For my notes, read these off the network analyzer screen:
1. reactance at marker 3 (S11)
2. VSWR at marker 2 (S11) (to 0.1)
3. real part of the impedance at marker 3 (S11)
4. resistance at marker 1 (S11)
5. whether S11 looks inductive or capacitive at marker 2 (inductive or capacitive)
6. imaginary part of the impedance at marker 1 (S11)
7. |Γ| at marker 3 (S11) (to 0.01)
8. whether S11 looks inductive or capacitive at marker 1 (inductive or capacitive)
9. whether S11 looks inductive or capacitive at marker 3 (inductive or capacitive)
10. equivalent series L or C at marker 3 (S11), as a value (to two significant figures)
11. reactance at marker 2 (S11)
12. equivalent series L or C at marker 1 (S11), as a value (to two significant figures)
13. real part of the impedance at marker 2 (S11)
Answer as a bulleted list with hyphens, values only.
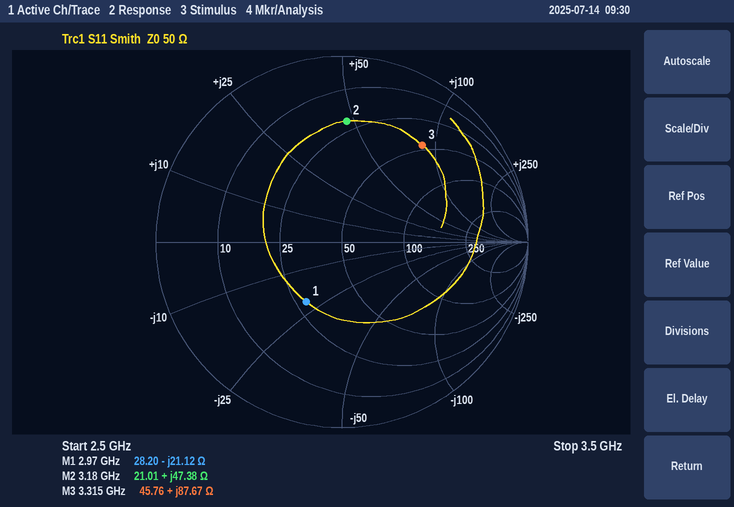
- +87.67 Ω
- 4.7
- 45.76 Ω
- 28.20 Ω
- inductive
- -21.12 Ω
- 0.68
- capacitive
- inductive
- 4.2 nH
- +47.38 Ω
- 2.5 pF
- 21.01 Ω
